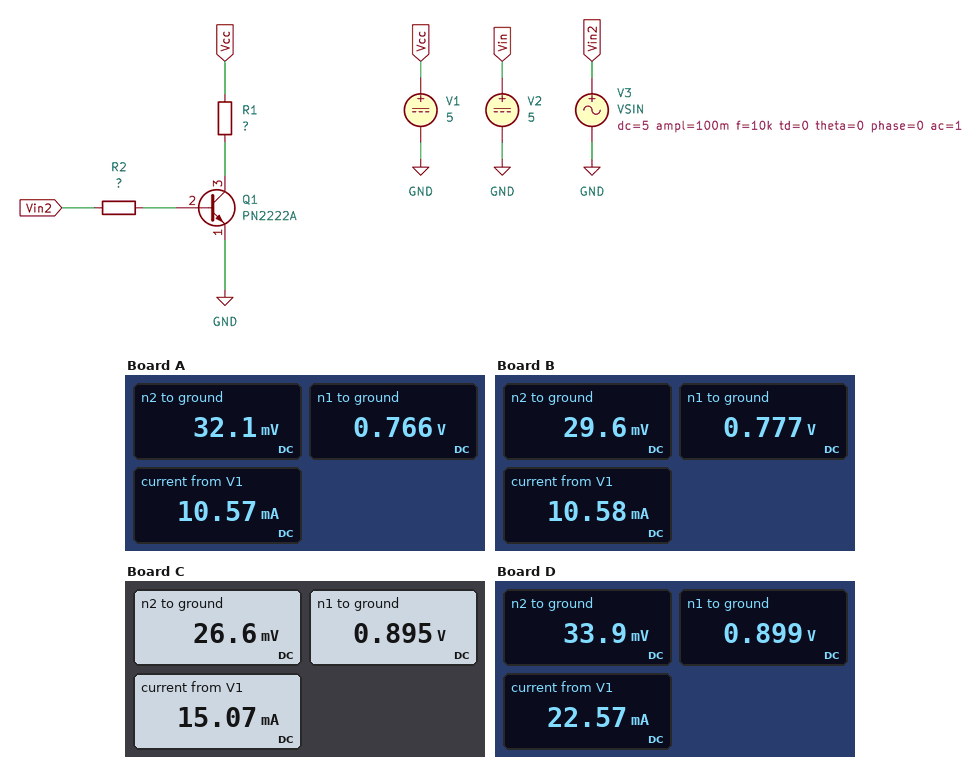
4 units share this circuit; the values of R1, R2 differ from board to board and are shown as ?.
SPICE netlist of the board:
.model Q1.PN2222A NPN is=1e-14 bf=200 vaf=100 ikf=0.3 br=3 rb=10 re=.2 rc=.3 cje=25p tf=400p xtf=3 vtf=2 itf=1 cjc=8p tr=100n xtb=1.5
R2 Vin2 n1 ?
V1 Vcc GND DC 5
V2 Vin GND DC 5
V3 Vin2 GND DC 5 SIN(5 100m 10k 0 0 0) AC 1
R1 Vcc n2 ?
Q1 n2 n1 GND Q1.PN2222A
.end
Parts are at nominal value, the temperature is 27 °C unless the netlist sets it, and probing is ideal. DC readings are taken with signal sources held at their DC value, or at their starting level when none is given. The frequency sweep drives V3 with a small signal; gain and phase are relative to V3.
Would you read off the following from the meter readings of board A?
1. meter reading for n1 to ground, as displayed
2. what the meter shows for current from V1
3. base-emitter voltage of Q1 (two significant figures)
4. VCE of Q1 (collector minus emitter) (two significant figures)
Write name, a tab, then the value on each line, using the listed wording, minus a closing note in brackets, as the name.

meter reading for n1 to ground, as displayed	0.766 V
what the meter shows for current from V1	10.57 mA
base-emitter voltage of Q1	770 mV
VCE of Q1 (collector minus emitter)	32 mV
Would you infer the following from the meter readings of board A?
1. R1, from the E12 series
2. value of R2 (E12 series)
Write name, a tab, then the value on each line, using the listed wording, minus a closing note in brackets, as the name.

R1, from the E12 series	470 Ω
value of R2	1.5 kΩ
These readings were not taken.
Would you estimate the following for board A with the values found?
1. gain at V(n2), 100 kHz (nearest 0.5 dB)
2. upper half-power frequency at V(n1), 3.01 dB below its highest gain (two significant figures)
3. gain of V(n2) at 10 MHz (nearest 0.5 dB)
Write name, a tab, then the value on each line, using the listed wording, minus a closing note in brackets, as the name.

gain at V(n2), 100 kHz	-51.0 dB
upper half-power frequency at V(n1), 3.01 dB below its highest gain	570 MHz
gain of V(n2) at 10 MHz	-60.0 dB
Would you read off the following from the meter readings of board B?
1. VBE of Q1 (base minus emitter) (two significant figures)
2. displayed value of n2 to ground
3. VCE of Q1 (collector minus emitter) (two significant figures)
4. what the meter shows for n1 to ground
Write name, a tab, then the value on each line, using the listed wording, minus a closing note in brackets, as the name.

VBE of Q1 (base minus emitter)	780 mV
displayed value of n2 to ground	29.6 mV
VCE of Q1 (collector minus emitter)	30 mV
what the meter shows for n1 to ground	0.777 V
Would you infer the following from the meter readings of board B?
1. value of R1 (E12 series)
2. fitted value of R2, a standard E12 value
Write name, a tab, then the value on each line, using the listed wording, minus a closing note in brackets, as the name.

value of R1	470 Ω
fitted value of R2, a standard E12 value	1.2 kΩ
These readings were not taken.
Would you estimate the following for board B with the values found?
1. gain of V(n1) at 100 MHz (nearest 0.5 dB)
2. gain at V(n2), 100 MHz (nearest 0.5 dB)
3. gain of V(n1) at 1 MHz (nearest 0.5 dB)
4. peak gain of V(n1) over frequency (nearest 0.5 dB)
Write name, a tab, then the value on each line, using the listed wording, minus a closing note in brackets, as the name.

gain of V(n1) at 100 MHz	-40.5 dB
gain at V(n2), 100 MHz	-59.5 dB
gain of V(n1) at 1 MHz	-40.0 dB
peak gain of V(n1) over frequency	-38.5 dB
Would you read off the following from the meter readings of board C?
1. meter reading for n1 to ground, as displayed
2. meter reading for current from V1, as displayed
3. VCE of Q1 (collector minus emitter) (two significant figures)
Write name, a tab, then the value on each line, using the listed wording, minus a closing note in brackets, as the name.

meter reading for n1 to ground, as displayed	0.895 V
meter reading for current from V1, as displayed	15.07 mA
VCE of Q1 (collector minus emitter)	27 mV
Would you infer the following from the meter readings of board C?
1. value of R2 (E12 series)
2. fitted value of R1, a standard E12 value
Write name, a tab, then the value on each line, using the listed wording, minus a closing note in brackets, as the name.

value of R2	330 Ω
fitted value of R1, a standard E12 value	330 Ω
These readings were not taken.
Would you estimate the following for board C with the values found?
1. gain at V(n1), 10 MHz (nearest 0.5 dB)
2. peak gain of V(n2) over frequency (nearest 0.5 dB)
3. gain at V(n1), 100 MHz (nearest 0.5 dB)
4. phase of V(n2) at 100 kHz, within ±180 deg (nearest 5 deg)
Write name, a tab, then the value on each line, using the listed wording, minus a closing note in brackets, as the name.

gain at V(n1), 10 MHz	-30.0 dB
peak gain of V(n2) over frequency	-54.0 dB
gain at V(n1), 100 MHz	-30.0 dB
phase of V(n2) at 100 kHz, within ±180 deg	140 deg
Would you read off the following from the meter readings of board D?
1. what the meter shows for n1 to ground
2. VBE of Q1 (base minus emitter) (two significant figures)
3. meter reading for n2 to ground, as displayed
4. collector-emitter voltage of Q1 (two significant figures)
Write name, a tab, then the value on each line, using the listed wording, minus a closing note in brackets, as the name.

what the meter shows for n1 to ground	0.899 V
VBE of Q1 (base minus emitter)	900 mV
meter reading for n2 to ground, as displayed	33.9 mV
collector-emitter voltage of Q1	34 mV
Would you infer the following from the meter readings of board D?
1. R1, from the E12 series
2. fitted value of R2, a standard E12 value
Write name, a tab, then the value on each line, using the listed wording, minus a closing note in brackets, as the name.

R1, from the E12 series	220 Ω
fitted value of R2, a standard E12 value	330 Ω
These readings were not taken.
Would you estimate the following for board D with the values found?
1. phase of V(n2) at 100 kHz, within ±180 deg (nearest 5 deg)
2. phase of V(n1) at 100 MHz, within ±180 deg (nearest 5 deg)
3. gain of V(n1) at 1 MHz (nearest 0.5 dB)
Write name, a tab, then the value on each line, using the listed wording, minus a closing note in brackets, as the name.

phase of V(n2) at 100 kHz, within ±180 deg	155 deg
phase of V(n1) at 100 MHz, within ±180 deg	0 deg
gain of V(n1) at 1 MHz	-30.0 dB
